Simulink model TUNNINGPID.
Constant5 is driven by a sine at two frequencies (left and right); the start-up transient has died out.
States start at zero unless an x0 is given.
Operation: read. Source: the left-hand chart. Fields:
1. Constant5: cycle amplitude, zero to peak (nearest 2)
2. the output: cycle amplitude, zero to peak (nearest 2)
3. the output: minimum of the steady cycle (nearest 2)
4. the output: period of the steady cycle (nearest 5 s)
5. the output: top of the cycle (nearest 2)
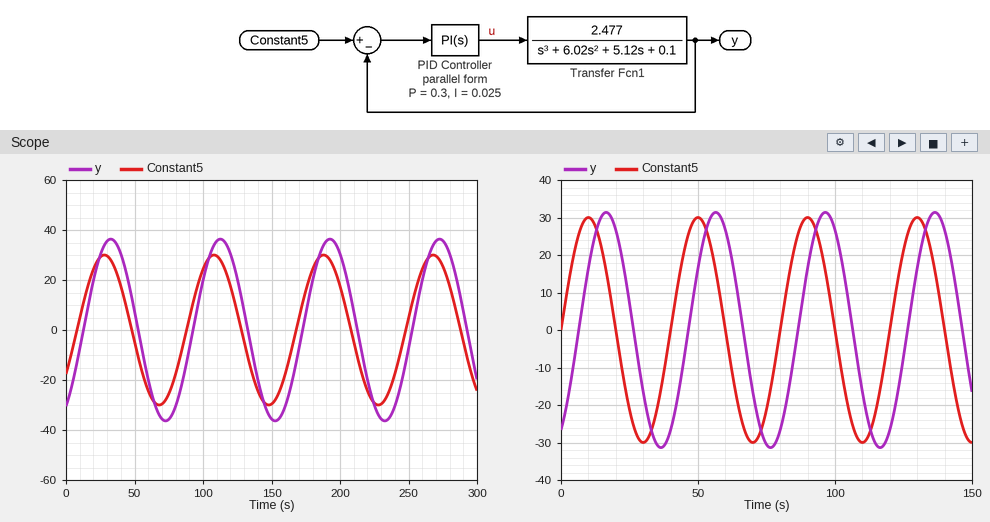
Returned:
30
36
-36
80 s
36
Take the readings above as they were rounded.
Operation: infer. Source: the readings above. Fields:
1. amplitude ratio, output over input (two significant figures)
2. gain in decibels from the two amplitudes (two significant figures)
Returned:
1.2
1.6 dB
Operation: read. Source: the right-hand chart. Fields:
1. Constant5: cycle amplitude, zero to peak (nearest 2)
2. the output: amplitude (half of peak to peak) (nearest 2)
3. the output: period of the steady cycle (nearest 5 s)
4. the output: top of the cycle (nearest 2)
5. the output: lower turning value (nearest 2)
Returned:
30
32
40 s
32
-32
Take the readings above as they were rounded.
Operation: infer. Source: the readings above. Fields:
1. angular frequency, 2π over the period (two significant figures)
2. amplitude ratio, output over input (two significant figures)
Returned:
0.16 rad/s
1.1
